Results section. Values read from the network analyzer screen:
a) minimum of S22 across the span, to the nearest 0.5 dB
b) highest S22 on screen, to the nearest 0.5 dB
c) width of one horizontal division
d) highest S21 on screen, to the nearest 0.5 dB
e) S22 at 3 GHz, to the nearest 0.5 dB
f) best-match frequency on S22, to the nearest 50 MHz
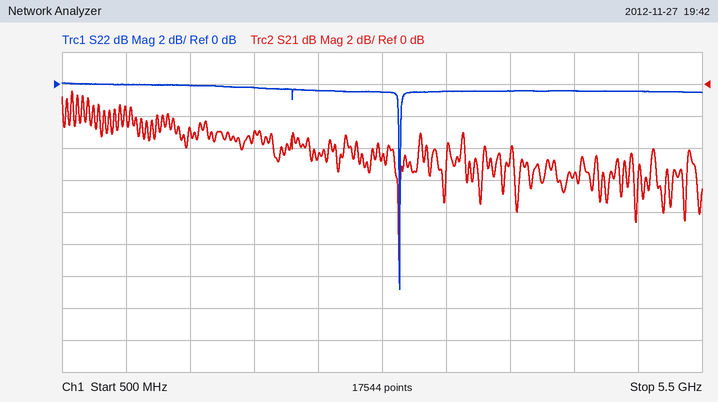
-13.0 dB
0.0 dB
500 MHz
-0.5 dB
-0.5 dB
3.15 GHz
